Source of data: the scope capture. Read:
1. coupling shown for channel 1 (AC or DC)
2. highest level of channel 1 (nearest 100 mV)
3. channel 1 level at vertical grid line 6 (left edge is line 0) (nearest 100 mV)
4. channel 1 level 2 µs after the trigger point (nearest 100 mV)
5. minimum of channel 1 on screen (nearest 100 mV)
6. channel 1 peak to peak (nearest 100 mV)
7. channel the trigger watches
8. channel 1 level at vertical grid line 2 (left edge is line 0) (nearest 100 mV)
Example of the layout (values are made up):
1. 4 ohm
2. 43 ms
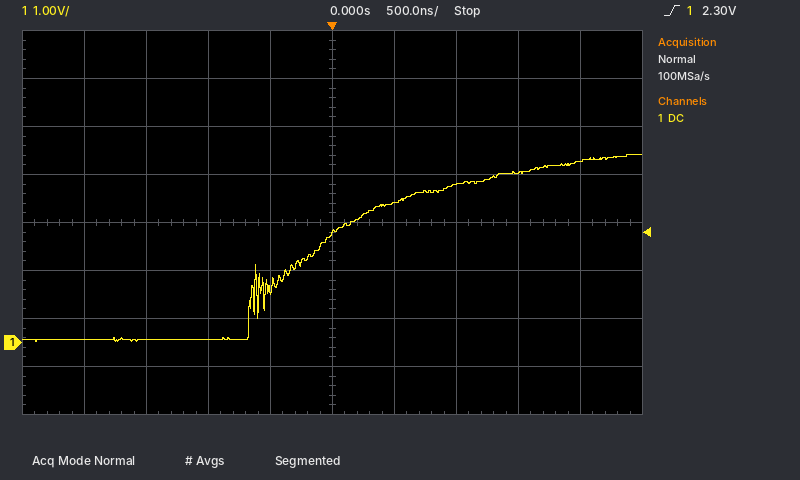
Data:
1. DC
2. 3.9 V
3. 2.9 V
4. 3.8 V
5. 0.0 V
6. 3.9 V
7. channel 1
8. 100 mV
